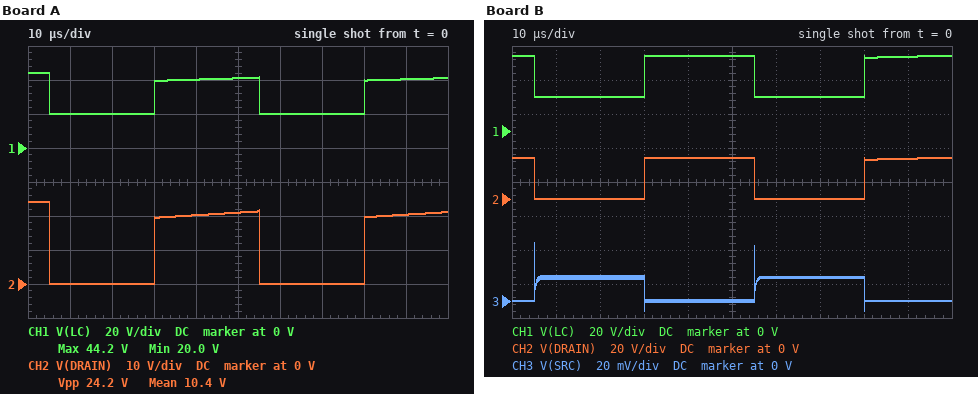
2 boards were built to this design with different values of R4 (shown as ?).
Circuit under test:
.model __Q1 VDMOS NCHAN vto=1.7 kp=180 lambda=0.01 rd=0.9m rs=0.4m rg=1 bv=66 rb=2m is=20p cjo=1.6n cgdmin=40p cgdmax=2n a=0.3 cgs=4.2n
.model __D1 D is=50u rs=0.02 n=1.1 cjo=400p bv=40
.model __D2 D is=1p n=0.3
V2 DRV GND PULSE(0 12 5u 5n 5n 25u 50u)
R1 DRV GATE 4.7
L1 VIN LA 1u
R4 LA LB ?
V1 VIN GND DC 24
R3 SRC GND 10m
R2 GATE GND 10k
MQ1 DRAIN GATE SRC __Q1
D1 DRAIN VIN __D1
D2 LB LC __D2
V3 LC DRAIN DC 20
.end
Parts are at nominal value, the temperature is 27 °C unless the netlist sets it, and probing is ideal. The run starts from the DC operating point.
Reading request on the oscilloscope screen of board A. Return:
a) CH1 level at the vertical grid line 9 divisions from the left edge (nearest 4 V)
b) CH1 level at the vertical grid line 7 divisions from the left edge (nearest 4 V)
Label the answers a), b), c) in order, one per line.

a) 40 V
b) 20 V
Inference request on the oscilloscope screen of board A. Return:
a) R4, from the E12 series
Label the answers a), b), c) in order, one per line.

a) 6.8 Ω
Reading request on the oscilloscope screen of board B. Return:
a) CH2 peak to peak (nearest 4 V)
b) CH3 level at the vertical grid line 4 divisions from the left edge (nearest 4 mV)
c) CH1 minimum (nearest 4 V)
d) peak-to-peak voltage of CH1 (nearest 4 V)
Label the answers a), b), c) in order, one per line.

a) 24 V
b) 0 V
c) 20 V
d) 24 V
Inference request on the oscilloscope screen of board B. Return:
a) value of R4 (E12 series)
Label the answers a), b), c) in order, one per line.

a) 2.7 Ω
